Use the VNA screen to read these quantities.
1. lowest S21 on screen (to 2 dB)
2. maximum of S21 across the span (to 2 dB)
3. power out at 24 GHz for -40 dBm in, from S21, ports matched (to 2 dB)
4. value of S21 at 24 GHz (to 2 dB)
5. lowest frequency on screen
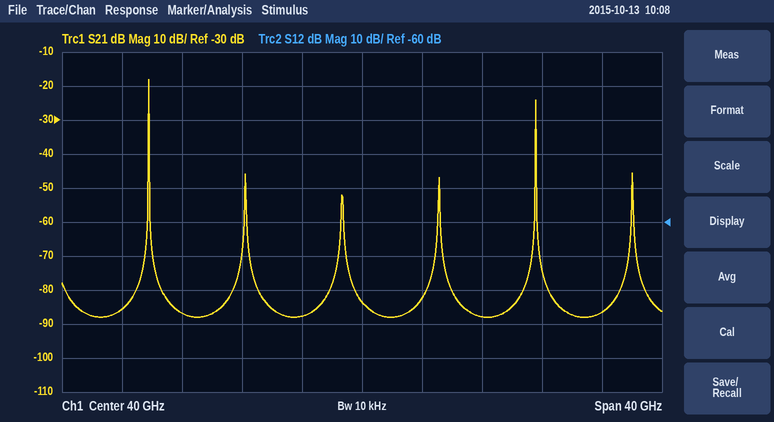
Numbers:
-88 dB
-18 dB
-126 dBm
-86 dB
20 GHz
